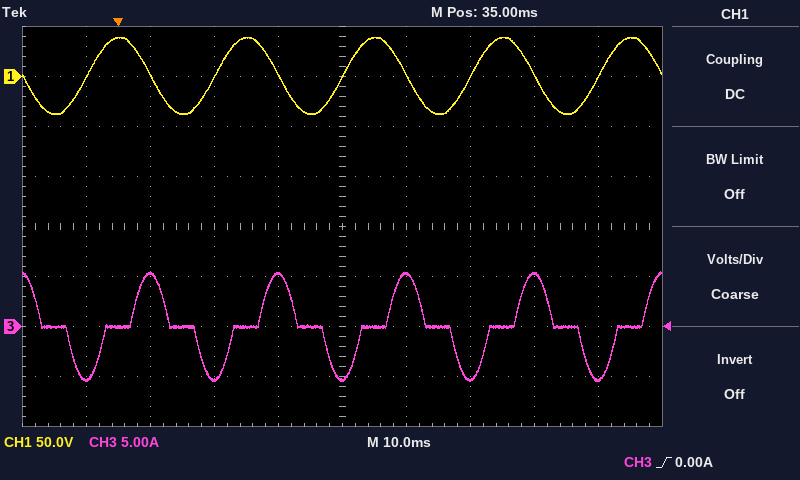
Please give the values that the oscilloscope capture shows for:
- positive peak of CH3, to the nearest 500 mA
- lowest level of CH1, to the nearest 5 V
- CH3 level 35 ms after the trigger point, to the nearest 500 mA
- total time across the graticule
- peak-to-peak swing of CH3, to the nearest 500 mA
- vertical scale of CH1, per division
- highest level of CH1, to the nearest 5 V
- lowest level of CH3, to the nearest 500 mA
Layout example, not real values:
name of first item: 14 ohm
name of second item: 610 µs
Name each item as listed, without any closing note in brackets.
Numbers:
positive peak of CH3, to the nearest 500 mA: 5.5 A
lowest level of CH1, to the nearest 5 V: -40 V
CH3 level 35 ms after the trigger point, to the nearest 500 mA: -5.5 A
total time across the graticule: 100 ms
peak-to-peak swing of CH3, to the nearest 500 mA: 11.0 A
vertical scale of CH1, per division: 50 V
highest level of CH1, to the nearest 5 V: 40 V
lowest level of CH3, to the nearest 500 mA: -5.5 A
